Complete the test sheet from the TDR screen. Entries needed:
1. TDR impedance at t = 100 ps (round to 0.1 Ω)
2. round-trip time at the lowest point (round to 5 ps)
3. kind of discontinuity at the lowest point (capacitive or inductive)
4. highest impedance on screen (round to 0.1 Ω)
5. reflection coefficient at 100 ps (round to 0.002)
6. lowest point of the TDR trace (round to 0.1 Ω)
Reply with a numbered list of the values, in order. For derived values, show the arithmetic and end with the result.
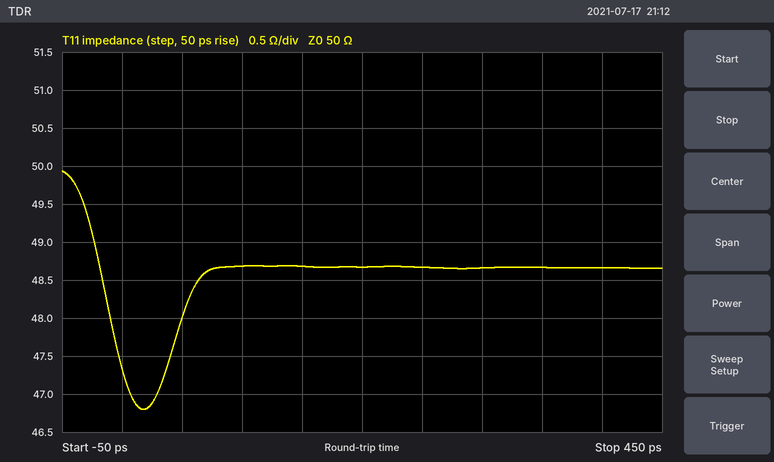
1. 48.7 Ω
2. 20 ps
3. capacitive
4. 49.9 Ω
5. (48.7 − 50)/(48.7 + 50) ≈ -0.0132, so -0.014 to the nearest 0.002
6. 46.8 Ω
